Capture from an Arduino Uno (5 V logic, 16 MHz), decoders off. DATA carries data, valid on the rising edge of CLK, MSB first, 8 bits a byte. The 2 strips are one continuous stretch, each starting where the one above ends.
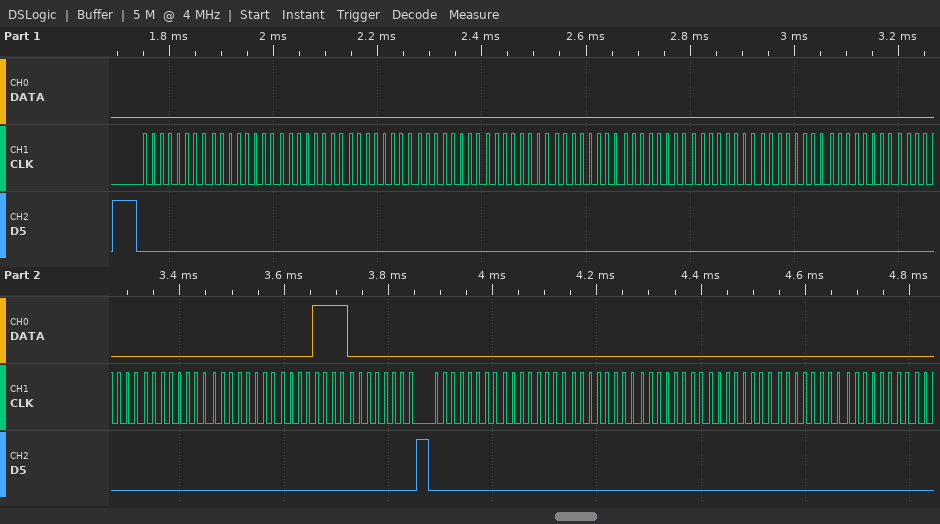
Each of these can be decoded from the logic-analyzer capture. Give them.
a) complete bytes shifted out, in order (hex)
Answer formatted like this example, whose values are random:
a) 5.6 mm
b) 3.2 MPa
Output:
a) 0x00 0x00 0x00 0x00 0x00 0x00 0x00 0x00 0x00 0x00 0x00 0x00 0x00 0x00 0x0F 0x00 0x00 0x00 0x00 0x00 0x00 0x00 0x00
